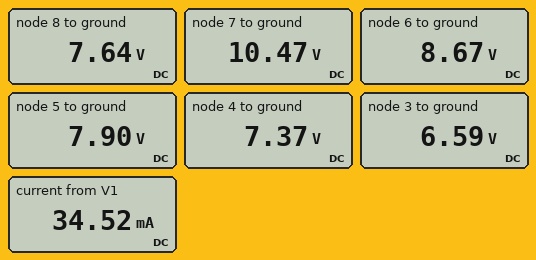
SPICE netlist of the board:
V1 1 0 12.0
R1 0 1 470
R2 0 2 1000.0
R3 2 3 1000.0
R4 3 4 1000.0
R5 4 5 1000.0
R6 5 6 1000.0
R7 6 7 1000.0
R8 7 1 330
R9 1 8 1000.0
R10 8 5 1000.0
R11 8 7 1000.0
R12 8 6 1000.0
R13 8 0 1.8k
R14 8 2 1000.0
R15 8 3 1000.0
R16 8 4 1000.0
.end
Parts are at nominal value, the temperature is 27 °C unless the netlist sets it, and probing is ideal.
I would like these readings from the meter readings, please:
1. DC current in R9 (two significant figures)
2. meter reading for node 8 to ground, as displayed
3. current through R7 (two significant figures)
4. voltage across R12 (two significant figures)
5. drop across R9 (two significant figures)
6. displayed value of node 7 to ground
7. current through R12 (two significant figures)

4.4 mA
7.64 V
1.8 mA
1.0 V
4.4 V
10.47 V
1.0 mA
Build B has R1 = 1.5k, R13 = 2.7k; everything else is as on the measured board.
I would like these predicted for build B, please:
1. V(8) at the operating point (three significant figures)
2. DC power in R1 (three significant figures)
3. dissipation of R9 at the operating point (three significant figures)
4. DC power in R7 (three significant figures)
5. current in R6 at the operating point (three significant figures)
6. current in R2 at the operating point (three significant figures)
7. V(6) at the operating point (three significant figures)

8.11 V
96.0 mW
15.1 mW
2.61 mW
709 µA
5.03 mA
9.02 V
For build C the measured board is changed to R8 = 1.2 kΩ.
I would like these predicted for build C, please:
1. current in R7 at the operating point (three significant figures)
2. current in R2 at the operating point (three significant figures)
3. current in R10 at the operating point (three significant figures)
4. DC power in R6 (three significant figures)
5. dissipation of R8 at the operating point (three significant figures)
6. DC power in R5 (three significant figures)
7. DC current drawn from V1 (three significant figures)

1.12 mA
4.23 mA
111 µA
255 µW
9.81 mW
155 µW
33.6 mA
